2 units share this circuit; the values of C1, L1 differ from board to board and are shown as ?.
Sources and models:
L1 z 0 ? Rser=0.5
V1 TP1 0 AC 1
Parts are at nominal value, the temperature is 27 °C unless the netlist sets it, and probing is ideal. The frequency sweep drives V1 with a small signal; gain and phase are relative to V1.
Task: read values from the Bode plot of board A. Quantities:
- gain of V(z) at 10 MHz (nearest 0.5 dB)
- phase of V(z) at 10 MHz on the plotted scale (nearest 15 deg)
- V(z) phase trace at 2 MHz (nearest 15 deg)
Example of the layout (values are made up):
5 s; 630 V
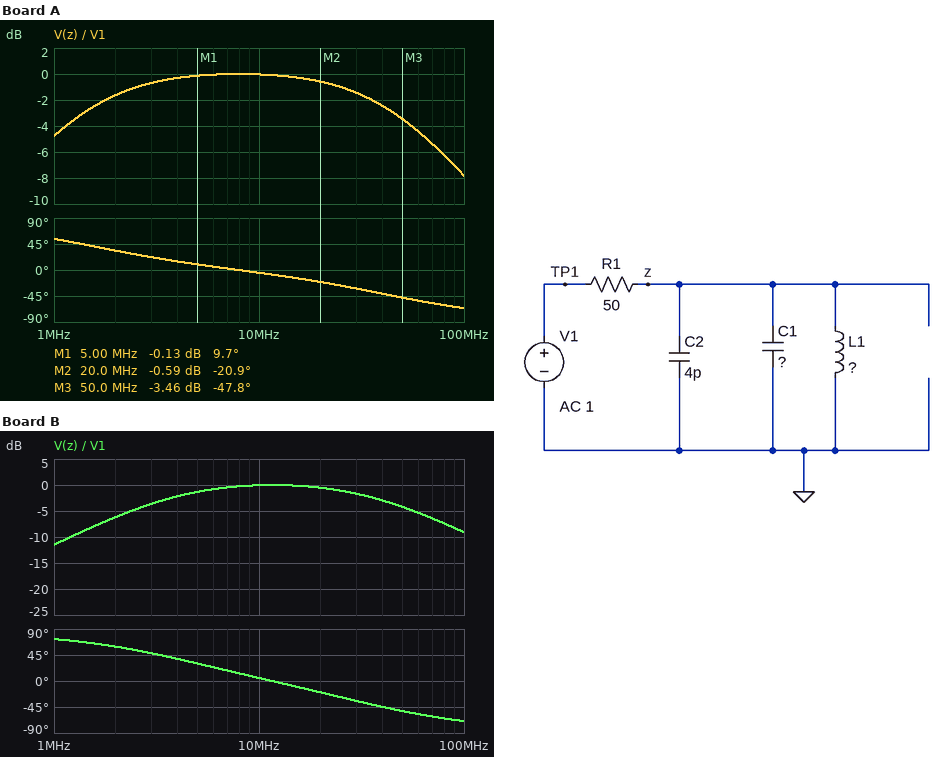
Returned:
0 dB; 0 deg; 30 deg
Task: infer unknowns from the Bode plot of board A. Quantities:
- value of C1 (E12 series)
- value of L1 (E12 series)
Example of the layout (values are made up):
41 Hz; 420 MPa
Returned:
68 pF; 5.6 µH
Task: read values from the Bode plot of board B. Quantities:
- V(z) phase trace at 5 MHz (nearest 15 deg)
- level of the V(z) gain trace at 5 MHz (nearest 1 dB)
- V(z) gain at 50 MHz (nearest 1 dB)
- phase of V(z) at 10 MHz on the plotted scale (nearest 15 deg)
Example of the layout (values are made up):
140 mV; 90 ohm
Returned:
30 deg; -1 dB; -4 dB; 0 deg
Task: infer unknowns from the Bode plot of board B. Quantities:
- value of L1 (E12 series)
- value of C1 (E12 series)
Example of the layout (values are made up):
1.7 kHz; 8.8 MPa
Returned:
2.2 µH; 82 pF
